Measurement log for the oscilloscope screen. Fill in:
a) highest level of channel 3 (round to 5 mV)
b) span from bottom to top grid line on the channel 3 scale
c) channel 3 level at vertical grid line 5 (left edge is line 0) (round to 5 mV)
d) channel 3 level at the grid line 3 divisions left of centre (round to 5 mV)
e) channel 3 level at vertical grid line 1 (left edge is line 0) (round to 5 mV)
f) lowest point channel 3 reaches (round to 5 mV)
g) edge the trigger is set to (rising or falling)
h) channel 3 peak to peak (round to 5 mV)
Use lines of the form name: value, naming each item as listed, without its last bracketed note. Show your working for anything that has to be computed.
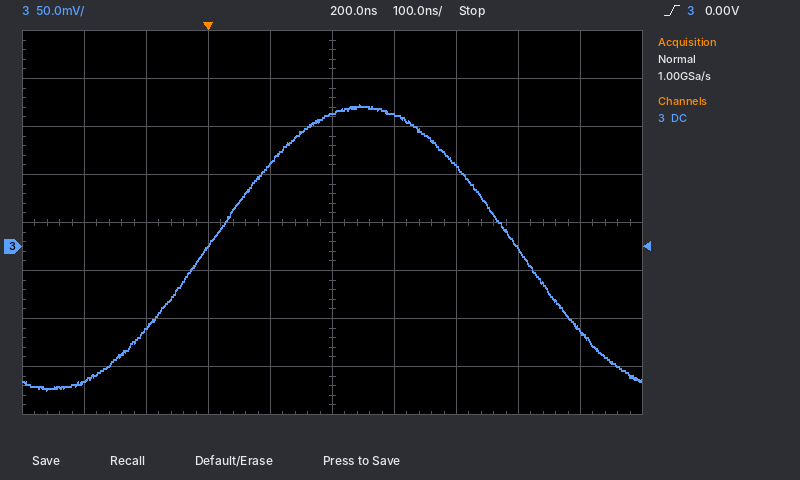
highest level of channel 3: 150 mV
span from bottom to top grid line on the channel 3 scale: 400 mV
channel 3 level at vertical grid line 5 (left edge is line 0): 140 mV
channel 3 level at the grid line 3 divisions left of centre: -85 mV
channel 3 level at vertical grid line 1 (left edge is line 0): -140 mV
lowest point channel 3 reaches: -150 mV
edge the trigger is set to: rising
channel 3 peak to peak: 150 mV − (-150 mV) = 300 mV
